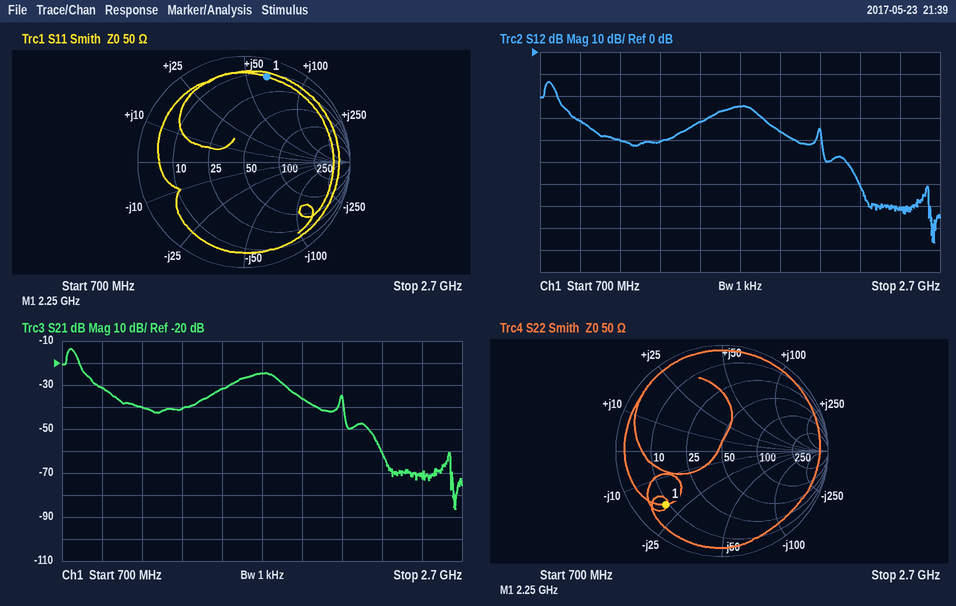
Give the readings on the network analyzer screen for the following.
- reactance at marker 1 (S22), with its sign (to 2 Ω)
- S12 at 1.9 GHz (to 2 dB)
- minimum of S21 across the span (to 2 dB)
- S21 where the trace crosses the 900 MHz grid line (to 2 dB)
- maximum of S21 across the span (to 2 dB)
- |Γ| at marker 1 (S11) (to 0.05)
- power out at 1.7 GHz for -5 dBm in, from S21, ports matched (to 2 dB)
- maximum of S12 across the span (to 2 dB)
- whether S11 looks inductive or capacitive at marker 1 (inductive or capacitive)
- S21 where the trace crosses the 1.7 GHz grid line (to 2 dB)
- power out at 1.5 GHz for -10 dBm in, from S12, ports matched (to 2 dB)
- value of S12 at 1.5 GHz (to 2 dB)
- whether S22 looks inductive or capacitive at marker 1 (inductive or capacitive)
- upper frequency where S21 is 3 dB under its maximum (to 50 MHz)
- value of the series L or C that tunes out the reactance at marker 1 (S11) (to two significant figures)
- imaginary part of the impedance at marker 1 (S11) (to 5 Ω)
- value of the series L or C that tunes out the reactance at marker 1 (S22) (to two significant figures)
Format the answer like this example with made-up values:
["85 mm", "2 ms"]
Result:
["-20 Ω", "-36 dB", "-86 dB", "-32 dB", "-14 dB", "0.85", "-30 dBm", "-14 dB", "inductive", "-24 dB", "-42 dBm", "-32 dB", "capacitive", "750 MHz", "1.1 pF", "+65 Ω", "1.4 nH"]
